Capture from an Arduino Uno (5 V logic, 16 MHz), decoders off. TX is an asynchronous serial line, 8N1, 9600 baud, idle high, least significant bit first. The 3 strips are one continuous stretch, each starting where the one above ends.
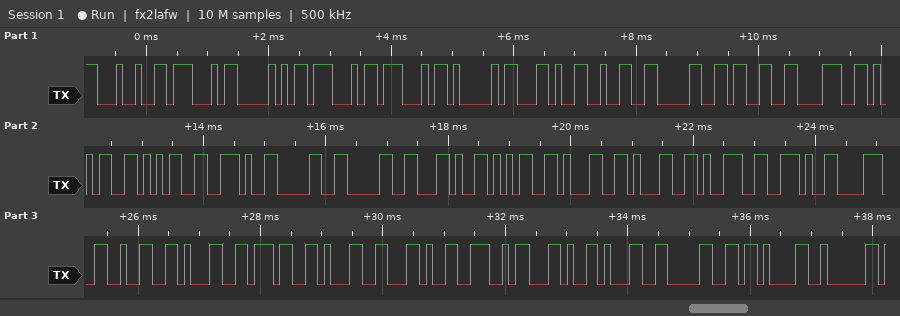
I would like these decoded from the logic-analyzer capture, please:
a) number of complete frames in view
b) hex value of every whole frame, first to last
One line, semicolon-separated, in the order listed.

34; 24 47 50 47 47 41 2C 32 30 33 38 35 35 2E 30 30 2C 35 31 31 39 2E 38 32 31 37 31 2C 4E 2C 31 30 0B 02
